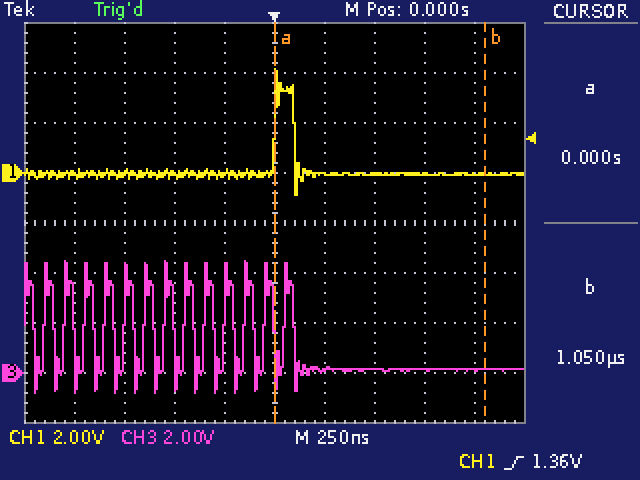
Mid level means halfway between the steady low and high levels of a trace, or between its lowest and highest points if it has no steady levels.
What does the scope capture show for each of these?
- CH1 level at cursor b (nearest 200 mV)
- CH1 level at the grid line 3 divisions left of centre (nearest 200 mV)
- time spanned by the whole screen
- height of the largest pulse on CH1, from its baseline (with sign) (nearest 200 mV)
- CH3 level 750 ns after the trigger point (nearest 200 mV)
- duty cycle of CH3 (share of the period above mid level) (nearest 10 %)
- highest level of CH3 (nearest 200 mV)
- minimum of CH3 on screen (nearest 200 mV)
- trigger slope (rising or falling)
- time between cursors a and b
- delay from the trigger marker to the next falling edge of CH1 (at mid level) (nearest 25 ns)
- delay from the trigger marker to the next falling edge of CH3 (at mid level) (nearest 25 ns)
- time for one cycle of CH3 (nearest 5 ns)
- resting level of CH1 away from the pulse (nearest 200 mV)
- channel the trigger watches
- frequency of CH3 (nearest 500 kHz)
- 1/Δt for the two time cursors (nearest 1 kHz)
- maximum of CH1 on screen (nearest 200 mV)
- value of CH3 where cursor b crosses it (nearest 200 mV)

0.0 V
0.0 V
2.5 µs
+4.2 V
200 mV
50 %
4.4 V
-800 mV
rising
1.050 µs
100 ns
100 ns
100 ns
0.0 V
CH1
10.0 MHz
952 kHz
4.2 V
200 mV
